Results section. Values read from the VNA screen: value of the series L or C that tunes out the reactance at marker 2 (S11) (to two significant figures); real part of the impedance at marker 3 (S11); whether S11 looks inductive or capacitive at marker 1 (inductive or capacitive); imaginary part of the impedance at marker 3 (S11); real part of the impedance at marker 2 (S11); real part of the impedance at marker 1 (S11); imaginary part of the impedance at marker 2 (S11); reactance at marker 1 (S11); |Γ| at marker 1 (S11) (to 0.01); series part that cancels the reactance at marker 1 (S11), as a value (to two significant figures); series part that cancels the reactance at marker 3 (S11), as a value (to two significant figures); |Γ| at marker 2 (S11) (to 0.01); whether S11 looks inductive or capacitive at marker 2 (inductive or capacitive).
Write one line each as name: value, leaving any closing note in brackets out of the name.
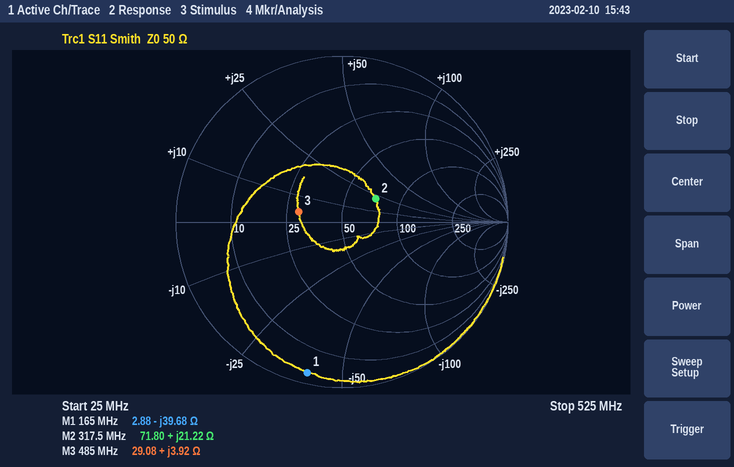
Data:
value of the series L or C that tunes out the reactance at marker 2 (S11): 24 pF
real part of the impedance at marker 3: 29.08 Ω
whether S11 looks inductive or capacitive at marker 1: capacitive
imaginary part of the impedance at marker 3: +3.92 Ω
real part of the impedance at marker 2: 71.80 Ω
real part of the impedance at marker 1: 2.88 Ω
imaginary part of the impedance at marker 2: +21.22 Ω
reactance at marker 1: -39.68 Ω
|Γ| at marker 1 (S11): 0.93
series part that cancels the reactance at marker 1 (S11), as a value: 38 nH
series part that cancels the reactance at marker 3 (S11), as a value: 84 pF
|Γ| at marker 2 (S11): 0.25
whether S11 looks inductive or capacitive at marker 2: inductive
